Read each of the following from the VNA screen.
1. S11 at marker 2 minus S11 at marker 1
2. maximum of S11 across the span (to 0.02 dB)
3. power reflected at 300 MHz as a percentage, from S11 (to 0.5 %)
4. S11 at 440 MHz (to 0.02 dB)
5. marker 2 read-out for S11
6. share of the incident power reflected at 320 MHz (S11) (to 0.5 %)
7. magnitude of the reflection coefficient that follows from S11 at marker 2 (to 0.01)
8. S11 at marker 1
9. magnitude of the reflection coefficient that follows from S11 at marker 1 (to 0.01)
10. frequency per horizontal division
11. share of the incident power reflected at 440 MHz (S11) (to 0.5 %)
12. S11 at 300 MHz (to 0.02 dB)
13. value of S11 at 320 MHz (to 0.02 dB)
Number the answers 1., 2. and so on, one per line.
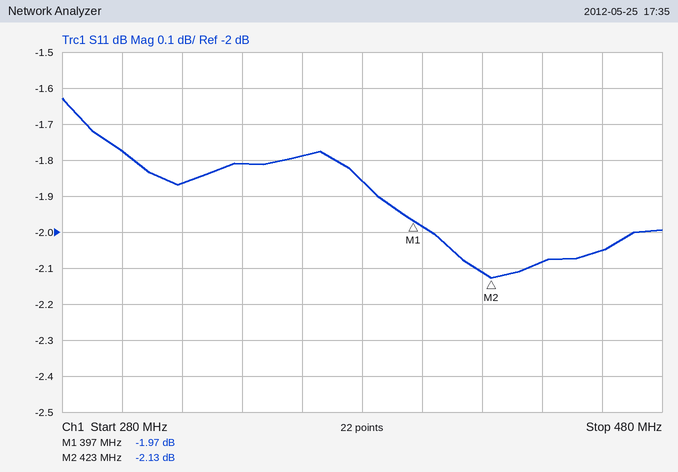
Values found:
1. -0.16 dB
2. -1.62 dB
3. 66.5 %
4. -2.08 dB
5. -2.13 dB
6. 65.0 %
7. 0.78
8. -1.97 dB
9. 0.80
10. 20 MHz
11. 62.0 %
12. -1.78 dB
13. -1.86 dB
